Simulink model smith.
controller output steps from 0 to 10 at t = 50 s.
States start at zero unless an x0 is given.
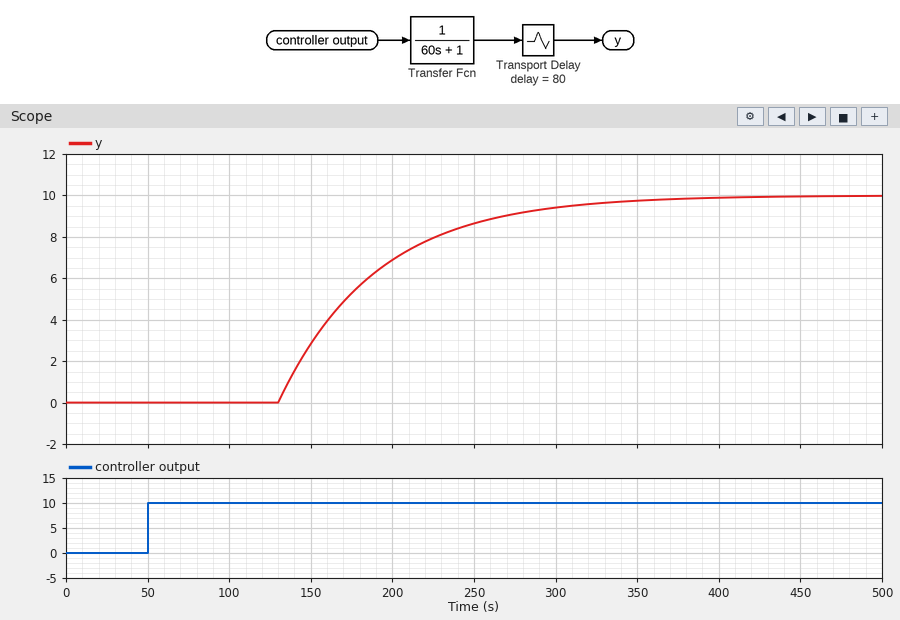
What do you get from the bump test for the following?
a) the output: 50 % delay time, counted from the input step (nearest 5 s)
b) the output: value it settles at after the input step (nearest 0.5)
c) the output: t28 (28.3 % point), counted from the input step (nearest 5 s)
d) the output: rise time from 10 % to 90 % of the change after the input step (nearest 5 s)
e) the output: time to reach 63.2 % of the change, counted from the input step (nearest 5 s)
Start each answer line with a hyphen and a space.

- 120 s
- 10.0
- 100 s
- 130 s
- 140 s
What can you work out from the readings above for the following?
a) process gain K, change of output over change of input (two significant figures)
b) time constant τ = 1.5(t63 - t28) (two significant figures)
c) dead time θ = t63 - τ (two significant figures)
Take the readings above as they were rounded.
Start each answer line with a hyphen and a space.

- 1.0
- 60 s
- 80 s
